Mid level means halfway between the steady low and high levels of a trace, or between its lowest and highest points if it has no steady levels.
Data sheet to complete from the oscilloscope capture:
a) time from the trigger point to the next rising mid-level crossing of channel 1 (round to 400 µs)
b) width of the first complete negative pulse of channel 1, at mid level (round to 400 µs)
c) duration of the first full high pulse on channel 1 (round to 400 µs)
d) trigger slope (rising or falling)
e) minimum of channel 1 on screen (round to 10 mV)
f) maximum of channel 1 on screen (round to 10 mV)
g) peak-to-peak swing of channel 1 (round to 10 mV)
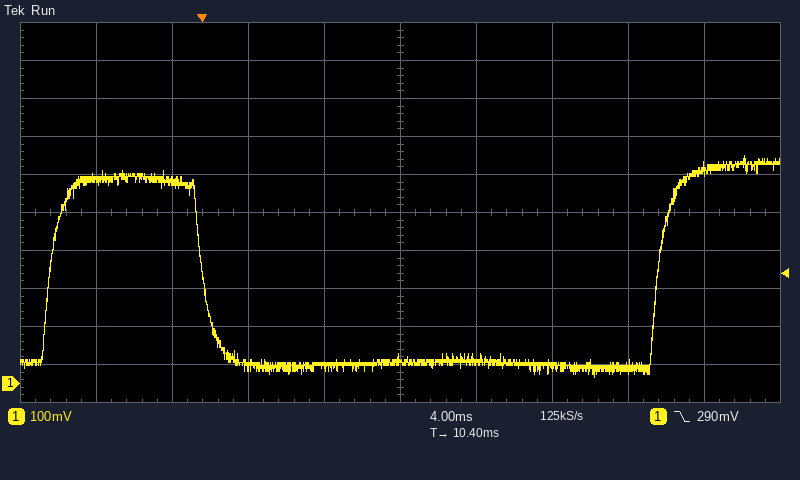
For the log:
24.0 ms
24.0 ms
8.0 ms
falling
20 mV
600 mV
580 mV
